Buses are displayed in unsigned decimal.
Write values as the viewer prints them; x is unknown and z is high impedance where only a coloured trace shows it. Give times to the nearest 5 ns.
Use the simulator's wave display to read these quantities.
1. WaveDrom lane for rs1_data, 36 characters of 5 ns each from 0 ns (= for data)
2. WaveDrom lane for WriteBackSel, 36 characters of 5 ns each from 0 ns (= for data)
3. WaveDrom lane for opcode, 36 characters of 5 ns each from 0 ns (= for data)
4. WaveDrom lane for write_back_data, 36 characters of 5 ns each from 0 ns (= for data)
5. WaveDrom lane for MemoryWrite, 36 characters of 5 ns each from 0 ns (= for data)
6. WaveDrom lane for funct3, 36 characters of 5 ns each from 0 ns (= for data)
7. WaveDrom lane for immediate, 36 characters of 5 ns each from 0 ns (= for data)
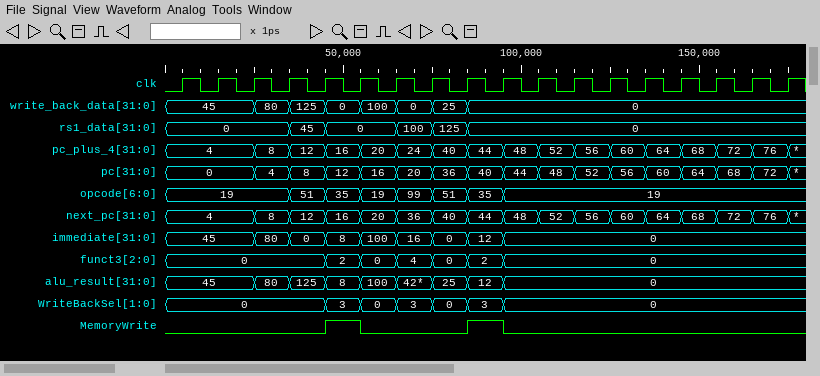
{name: 'rs1_data', wave: '=......=.=...=.=.=..................', data: '0 45 0 100 125 0'}
{name: 'WriteBackSel', wave: '=........=.=.=.=.=.=................', data: '0 3 0 3 0 3 0'}
{name: 'opcode', wave: '=......=.=.=.=.=.=.=................', data: '19 51 35 19 99 51 35 19'}
{name: 'write_back_data', wave: '=....=.=.=.=.=.=.=..................', data: '45 80 125 0 100 0 25 0'}
{name: 'MemoryWrite', wave: '0........1.0.....1.0................'}
{name: 'funct3', wave: '=........=.=.=.=.=.=................', data: '0 2 0 4 0 2 0'}
{name: 'immediate', wave: '=....=.=.=.=.=.=.=.=................', data: '45 80 0 8 100 16 0 12 0'}
